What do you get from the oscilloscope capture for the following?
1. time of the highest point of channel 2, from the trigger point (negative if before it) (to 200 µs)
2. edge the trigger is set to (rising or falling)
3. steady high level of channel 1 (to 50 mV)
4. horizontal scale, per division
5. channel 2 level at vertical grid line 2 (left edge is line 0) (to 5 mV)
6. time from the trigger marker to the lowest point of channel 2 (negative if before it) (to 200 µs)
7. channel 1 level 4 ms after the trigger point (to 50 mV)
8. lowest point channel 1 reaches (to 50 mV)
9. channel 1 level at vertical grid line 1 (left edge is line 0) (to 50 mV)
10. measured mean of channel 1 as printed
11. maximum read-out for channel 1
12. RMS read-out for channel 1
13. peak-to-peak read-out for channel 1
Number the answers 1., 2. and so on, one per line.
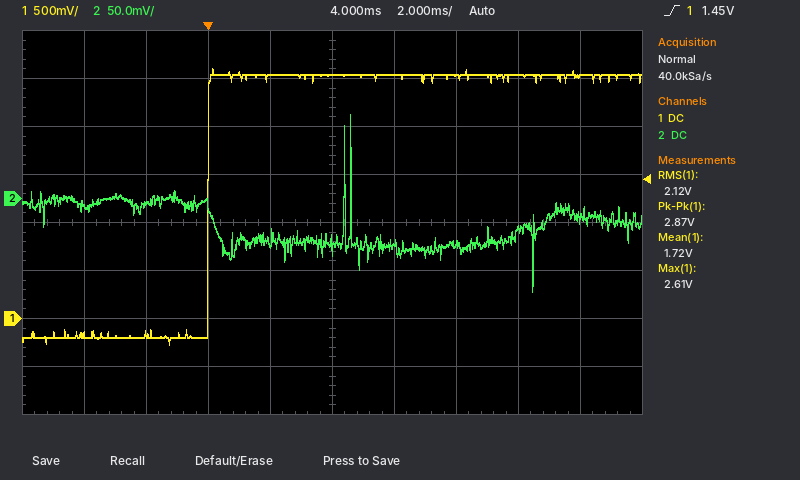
1. +4.6 ms
2. rising
3. 2.55 V
4. 2 ms
5. -5 mV
6. +10.4 ms
7. 2.55 V
8. -250 mV
9. -150 mV
10. 1.72 V
11. 2.61 V
12. 2.12 V
13. 2.87 V
